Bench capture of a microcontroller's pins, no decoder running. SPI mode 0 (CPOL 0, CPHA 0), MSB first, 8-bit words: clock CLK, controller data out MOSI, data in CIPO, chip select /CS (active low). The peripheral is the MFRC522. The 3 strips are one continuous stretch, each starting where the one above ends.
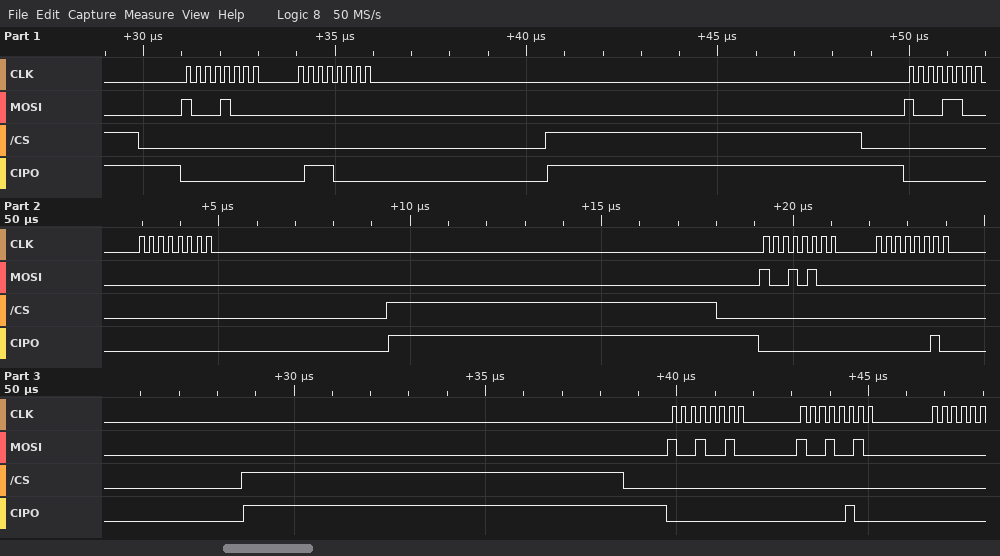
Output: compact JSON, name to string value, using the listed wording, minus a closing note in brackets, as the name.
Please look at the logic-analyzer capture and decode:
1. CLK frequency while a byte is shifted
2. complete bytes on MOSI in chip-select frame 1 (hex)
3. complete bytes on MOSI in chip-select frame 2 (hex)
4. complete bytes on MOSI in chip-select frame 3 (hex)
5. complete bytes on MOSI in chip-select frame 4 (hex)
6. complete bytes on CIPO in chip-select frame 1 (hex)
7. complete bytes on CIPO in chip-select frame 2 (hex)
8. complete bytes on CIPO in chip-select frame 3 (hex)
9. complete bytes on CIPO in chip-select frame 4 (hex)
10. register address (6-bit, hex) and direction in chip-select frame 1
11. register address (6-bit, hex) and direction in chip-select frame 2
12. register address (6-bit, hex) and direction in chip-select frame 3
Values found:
{"CLK frequency while a byte is shifted": "4 MHz", "complete bytes on MOSI in chip-select frame 1": "88 00", "complete bytes on MOSI in chip-select frame 2": "8C 00", "complete bytes on MOSI in chip-select frame 3": "94 00", "complete bytes on MOSI in chip-select frame 4": "92 92", "complete bytes on CIPO in chip-select frame 1": "00 70", "complete bytes on CIPO in chip-select frame 2": "00 00", "complete bytes on CIPO in chip-select frame 3": "00 02", "complete bytes on CIPO in chip-select frame 4": "00 04", "register address (6-bit, hex) and direction in chip-select frame 1": "0x04 read", "register address (6-bit, hex) and direction in chip-select frame 2": "0x06 read", "register address (6-bit, hex) and direction in chip-select frame 3": "0x0A read"}
